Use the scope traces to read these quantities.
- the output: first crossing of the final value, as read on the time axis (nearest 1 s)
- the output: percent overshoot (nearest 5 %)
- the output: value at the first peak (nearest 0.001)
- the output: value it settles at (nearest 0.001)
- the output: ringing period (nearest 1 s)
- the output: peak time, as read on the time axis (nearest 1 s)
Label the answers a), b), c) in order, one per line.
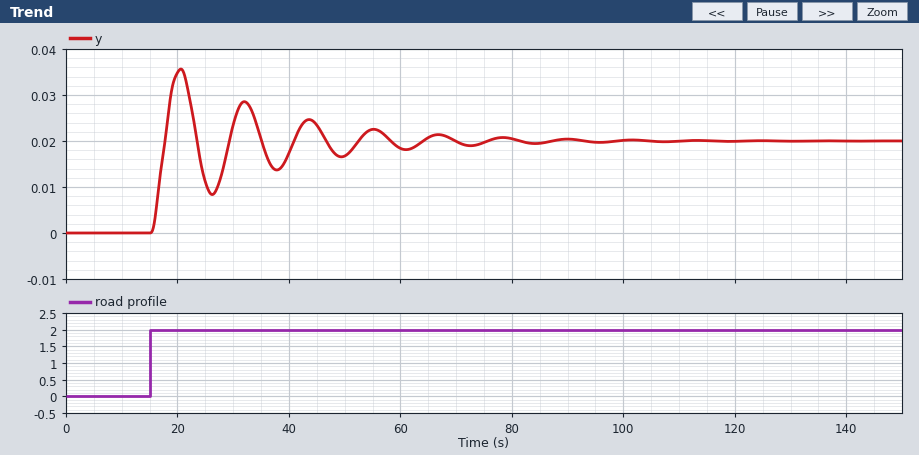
a) 18 s
b) 80 %
c) 0.036
d) 0.020
e) 11 s
f) 21 s
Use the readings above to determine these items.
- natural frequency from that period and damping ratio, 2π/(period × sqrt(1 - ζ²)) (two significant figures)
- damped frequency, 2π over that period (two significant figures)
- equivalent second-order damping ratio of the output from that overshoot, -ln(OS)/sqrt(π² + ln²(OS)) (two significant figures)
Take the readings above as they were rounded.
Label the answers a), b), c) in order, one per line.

a) 0.57 rad/s
b) 0.57 rad/s
c) 0.071
